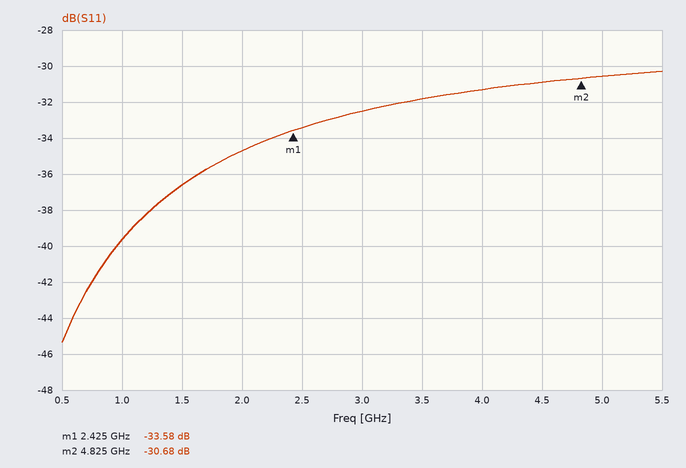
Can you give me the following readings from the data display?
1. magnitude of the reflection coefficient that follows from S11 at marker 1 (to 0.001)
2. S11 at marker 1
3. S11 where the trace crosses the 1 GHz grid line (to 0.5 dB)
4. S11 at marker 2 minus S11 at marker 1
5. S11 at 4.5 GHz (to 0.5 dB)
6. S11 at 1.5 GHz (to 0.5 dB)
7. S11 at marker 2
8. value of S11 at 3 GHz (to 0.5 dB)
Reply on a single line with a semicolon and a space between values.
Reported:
0.021; -33.58 dB; -39.5 dB; 2.90 dB; -31.0 dB; -36.5 dB; -30.68 dB; -32.5 dB
